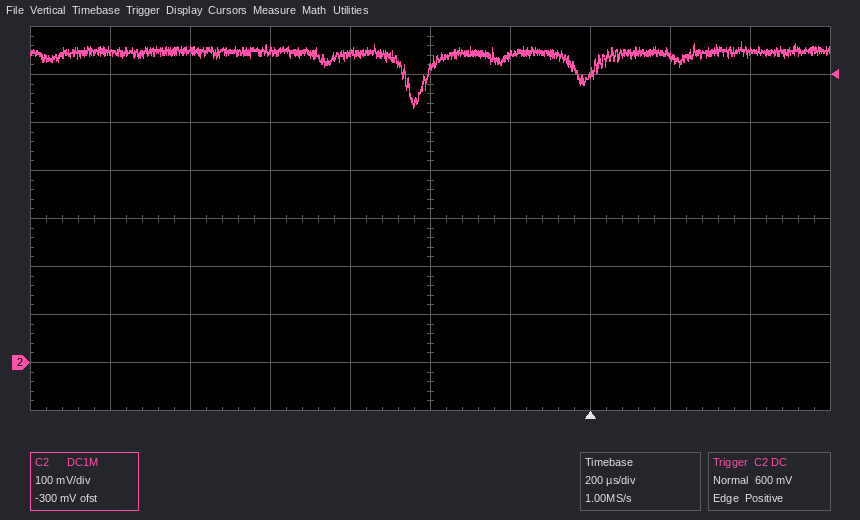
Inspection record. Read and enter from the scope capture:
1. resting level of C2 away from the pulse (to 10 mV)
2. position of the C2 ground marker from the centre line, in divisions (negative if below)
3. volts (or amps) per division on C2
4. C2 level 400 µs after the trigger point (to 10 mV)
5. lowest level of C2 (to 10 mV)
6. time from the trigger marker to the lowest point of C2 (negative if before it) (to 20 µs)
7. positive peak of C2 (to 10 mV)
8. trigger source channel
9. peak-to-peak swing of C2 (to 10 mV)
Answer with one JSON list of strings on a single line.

["650 mV", "-3.0 div", "100 mV", "650 mV", "530 mV", "-440 µs", "670 mV", "C2", "140 mV"]
